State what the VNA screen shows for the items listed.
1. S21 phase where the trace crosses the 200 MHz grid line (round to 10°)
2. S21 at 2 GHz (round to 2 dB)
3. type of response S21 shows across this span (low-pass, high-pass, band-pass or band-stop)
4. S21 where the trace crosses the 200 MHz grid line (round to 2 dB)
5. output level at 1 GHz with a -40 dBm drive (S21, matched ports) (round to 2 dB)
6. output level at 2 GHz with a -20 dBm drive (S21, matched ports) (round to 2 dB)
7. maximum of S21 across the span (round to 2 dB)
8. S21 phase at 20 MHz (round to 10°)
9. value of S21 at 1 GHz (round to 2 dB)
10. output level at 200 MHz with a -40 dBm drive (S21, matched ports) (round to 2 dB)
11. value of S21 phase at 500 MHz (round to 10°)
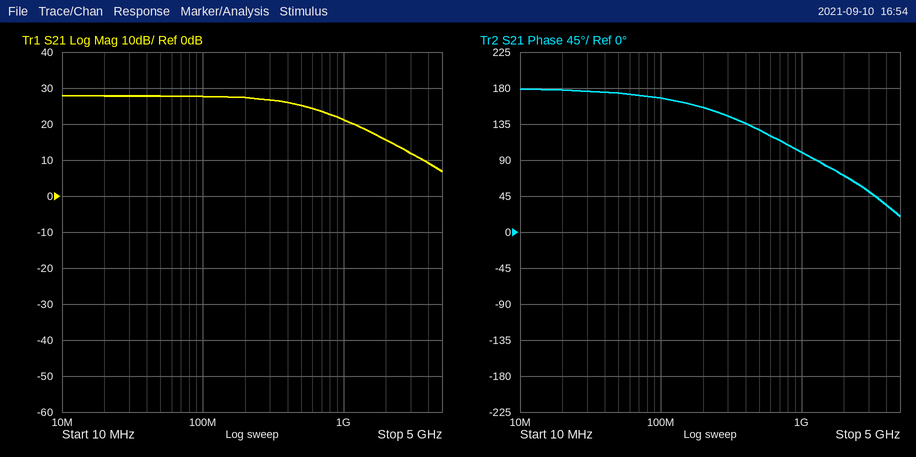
160°
16 dB
low-pass
28 dB
-18 dBm
-4 dBm
28 dB
180°
22 dB
-12 dBm
130°
